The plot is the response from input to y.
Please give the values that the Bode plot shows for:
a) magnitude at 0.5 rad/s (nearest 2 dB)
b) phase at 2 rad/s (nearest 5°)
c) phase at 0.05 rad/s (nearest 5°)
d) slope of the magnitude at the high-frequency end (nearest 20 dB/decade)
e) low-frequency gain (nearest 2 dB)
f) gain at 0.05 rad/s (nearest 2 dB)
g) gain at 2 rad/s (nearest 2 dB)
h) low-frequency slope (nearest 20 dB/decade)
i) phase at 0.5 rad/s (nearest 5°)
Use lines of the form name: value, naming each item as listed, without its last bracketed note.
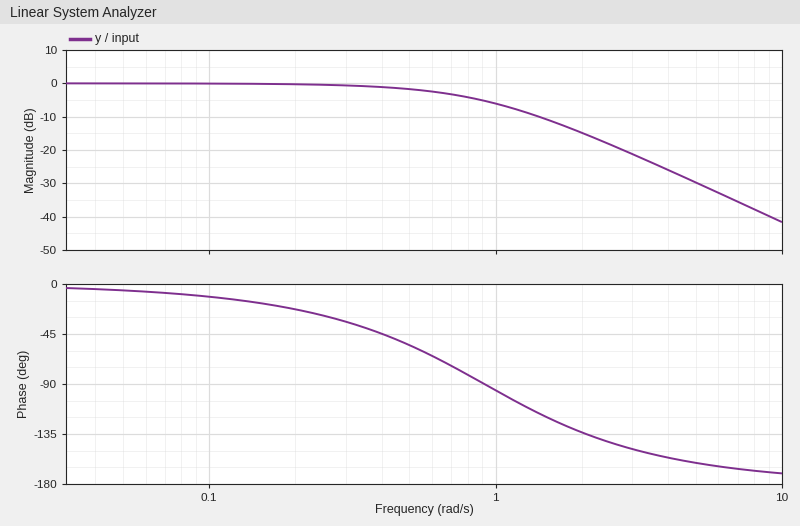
magnitude at 0.5 rad/s: -2 dB
phase at 2 rad/s: -135°
phase at 0.05 rad/s: -5°
slope of the magnitude at the high-frequency end: -40 dB/decade
low-frequency gain: 0 dB
gain at 0.05 rad/s: 0 dB
gain at 2 rad/s: -14 dB
low-frequency slope: 0 dB/decade
phase at 0.5 rad/s: -55°
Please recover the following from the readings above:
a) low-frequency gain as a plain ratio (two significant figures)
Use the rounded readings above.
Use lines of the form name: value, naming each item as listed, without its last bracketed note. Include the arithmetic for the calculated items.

low-frequency gain as a plain ratio: 10^(0 / 20) = 1.0
